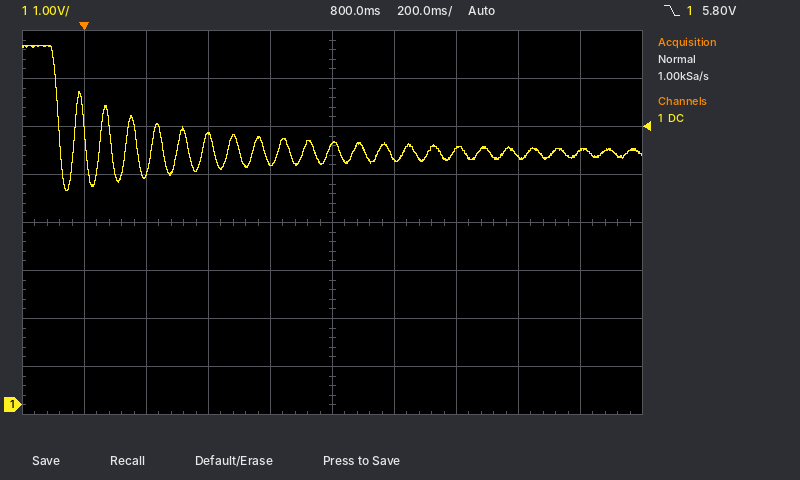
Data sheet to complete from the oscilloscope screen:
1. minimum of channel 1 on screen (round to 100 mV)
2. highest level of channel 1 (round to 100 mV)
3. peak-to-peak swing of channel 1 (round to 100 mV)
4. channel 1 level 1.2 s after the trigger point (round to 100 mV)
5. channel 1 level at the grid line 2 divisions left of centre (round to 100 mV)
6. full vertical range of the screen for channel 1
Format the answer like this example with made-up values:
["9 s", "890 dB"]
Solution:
["4.5 V", "7.5 V", "3.0 V", "5.3 V", "5.6 V", "8 V"]
